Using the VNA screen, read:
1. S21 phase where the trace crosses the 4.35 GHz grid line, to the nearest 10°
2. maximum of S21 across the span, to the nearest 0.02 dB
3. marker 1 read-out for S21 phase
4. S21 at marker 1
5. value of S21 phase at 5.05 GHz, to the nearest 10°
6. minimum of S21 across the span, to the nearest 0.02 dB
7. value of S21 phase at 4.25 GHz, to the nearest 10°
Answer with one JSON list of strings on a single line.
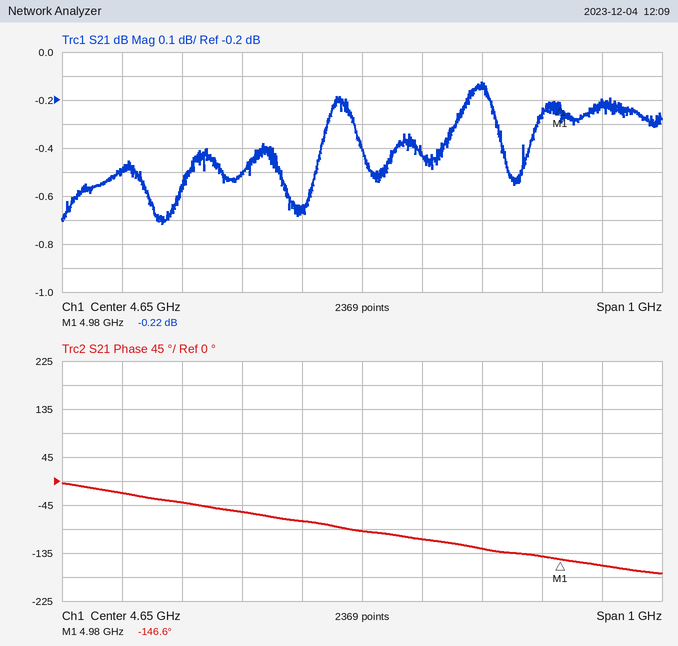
["-40°", "-0.12 dB", "-146.6°", "-0.22 dB", "-160°", "-0.72 dB", "-20°"]
